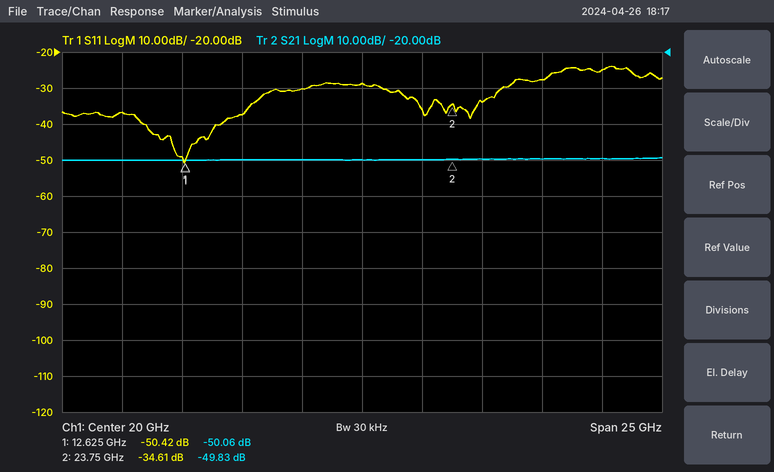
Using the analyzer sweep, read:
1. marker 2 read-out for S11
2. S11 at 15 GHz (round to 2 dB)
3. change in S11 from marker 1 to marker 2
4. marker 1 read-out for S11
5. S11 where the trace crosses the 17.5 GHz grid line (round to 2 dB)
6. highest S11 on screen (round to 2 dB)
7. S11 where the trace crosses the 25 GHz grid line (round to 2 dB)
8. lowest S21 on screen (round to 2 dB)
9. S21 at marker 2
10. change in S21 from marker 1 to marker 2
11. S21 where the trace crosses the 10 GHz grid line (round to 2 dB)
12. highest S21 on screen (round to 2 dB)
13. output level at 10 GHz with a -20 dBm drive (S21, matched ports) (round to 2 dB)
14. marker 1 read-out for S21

-34.61 dB
-38 dB
15.81 dB
-50.42 dB
-30 dB
-24 dB
-34 dB
-50 dB
-49.83 dB
0.23 dB
-50 dB
-50 dB
-70 dBm
-50.06 dB
